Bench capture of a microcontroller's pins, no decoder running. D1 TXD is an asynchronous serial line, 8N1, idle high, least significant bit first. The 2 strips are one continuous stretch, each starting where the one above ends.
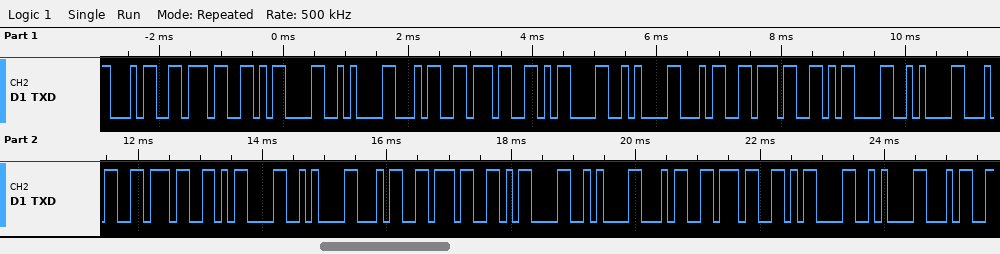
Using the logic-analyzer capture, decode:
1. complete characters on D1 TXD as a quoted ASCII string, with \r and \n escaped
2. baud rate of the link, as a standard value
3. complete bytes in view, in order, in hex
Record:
"47\r\n47\r\n47\r\n47\r\n47\r\n47\r\n4"
9600 baud
34 37 0D 0A 34 37 0D 0A 34 37 0D 0A 34 37 0D 0A 34 37 0D 0A 34 37 0D 0A 34
